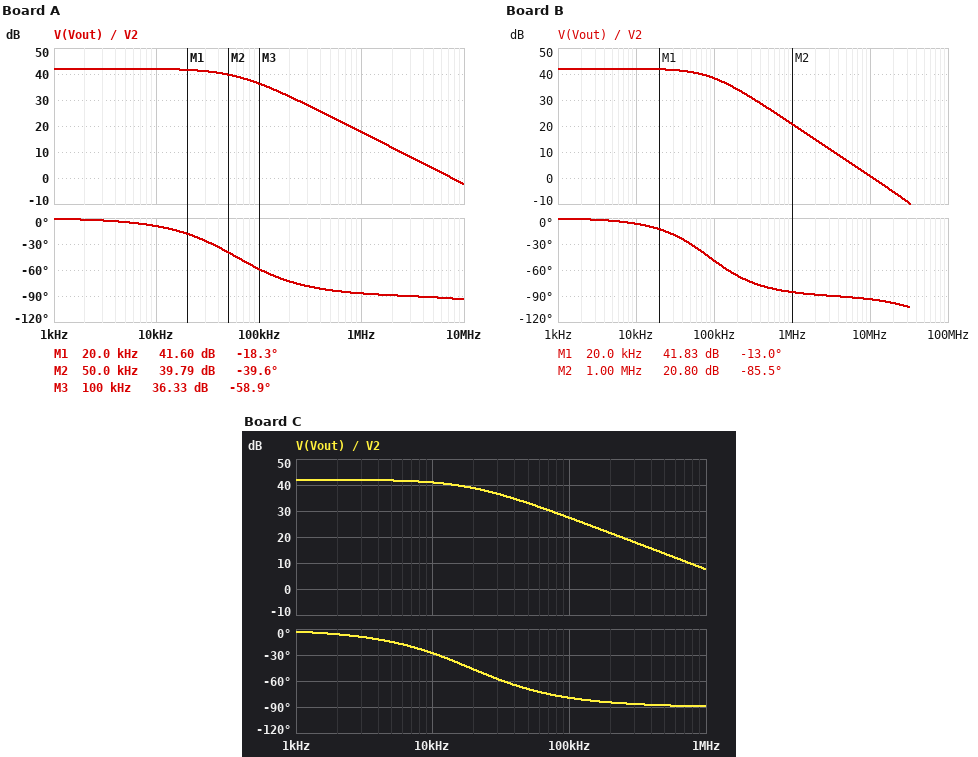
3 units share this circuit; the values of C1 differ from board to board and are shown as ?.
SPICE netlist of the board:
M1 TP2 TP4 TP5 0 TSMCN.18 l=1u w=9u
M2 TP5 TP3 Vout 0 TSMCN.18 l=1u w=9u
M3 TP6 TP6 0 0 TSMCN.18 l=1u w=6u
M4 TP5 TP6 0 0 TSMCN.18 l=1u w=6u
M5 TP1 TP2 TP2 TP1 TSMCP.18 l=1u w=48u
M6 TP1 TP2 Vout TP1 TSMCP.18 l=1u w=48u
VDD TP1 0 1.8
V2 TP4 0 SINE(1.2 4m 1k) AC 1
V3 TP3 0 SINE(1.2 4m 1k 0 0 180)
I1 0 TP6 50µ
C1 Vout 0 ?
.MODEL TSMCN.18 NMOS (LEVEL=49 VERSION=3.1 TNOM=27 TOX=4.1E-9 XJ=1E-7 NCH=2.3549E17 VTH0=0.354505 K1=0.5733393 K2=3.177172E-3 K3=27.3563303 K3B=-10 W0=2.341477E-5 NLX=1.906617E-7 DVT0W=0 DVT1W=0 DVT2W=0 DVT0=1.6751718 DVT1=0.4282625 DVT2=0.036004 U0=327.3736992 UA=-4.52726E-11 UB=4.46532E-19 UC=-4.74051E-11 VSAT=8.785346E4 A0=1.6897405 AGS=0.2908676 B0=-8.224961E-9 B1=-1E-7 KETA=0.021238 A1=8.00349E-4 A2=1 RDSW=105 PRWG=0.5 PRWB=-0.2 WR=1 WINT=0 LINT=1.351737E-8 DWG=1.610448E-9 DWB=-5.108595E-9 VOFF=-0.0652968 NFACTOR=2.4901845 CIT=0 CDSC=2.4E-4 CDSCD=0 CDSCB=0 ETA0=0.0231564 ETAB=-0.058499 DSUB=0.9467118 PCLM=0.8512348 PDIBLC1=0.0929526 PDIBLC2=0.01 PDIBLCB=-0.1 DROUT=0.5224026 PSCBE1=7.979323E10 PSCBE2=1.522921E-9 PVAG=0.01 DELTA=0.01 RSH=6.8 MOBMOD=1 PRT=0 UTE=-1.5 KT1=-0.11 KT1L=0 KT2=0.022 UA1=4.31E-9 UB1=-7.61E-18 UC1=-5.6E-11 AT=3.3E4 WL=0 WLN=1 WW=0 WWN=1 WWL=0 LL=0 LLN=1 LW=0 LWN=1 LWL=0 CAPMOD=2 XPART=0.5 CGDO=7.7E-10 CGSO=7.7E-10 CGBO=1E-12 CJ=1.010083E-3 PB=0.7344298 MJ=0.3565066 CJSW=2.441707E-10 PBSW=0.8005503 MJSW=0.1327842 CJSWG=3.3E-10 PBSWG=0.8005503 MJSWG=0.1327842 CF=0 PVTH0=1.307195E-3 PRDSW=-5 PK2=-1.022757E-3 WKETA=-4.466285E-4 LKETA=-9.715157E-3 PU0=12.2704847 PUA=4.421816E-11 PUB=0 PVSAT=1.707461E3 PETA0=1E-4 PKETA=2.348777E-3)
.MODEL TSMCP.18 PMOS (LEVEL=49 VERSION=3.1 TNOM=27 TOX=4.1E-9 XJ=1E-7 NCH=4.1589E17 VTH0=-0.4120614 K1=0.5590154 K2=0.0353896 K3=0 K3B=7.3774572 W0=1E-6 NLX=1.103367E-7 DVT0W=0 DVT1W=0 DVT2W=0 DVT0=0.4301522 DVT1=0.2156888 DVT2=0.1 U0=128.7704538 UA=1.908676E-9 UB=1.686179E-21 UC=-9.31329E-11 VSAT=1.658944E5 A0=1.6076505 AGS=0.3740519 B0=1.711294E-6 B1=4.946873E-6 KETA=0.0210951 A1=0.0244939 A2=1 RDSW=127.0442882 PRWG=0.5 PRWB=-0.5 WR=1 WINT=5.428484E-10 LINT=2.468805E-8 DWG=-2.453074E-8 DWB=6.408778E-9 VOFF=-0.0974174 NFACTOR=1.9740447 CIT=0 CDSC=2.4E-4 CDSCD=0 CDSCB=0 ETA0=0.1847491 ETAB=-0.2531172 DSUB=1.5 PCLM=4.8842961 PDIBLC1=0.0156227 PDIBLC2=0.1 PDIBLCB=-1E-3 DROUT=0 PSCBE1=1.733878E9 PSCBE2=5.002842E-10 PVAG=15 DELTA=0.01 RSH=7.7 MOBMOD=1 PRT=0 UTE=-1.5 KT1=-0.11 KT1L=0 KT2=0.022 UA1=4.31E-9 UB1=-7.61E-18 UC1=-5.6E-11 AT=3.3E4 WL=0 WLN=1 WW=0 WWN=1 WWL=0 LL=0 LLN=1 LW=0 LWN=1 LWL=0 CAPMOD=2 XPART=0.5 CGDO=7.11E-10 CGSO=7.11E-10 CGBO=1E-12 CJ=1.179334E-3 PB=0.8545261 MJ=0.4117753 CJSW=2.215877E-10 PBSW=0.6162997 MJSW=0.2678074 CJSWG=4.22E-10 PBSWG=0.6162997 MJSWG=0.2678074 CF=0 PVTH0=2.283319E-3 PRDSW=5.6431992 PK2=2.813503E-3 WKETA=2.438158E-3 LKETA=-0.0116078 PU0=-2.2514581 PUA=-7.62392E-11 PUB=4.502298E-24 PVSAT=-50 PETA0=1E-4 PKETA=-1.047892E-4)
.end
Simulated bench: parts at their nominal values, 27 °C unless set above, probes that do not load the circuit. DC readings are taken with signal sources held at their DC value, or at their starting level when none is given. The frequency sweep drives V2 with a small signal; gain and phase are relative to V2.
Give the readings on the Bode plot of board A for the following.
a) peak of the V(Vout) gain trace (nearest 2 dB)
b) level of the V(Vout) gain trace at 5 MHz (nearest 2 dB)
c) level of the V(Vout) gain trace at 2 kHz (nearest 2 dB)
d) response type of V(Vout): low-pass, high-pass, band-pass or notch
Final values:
42 dB
4 dB
42 dB
low-pass
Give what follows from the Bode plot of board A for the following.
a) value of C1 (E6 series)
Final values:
6.8 pF
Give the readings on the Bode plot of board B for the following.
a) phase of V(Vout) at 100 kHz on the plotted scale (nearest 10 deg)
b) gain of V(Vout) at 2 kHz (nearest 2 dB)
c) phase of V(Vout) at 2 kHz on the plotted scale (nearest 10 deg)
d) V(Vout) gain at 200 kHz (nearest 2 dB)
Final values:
-50 deg
42 dB
0 deg
34 dB
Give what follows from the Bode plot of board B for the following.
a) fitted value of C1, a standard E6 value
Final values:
4.7 pF
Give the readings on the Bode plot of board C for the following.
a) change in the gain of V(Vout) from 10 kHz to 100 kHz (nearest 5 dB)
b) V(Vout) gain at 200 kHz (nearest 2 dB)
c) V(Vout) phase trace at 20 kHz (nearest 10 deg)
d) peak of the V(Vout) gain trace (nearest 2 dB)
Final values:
-15 dB
22 dB
-50 deg
42 dB
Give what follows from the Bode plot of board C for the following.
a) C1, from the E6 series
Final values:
22 pF
